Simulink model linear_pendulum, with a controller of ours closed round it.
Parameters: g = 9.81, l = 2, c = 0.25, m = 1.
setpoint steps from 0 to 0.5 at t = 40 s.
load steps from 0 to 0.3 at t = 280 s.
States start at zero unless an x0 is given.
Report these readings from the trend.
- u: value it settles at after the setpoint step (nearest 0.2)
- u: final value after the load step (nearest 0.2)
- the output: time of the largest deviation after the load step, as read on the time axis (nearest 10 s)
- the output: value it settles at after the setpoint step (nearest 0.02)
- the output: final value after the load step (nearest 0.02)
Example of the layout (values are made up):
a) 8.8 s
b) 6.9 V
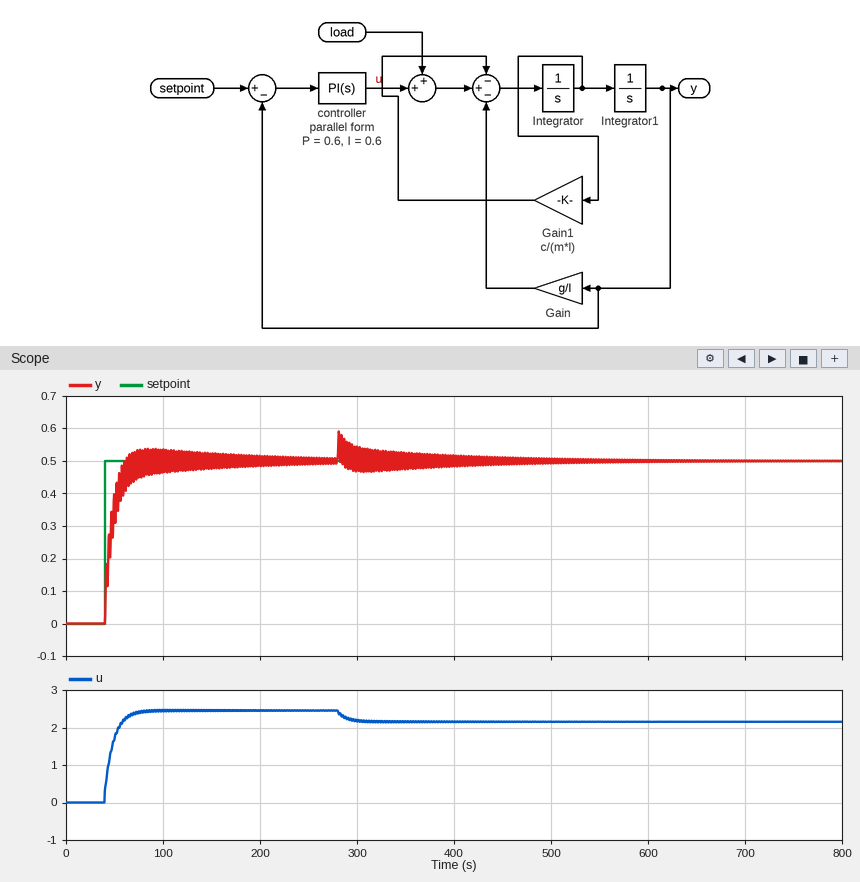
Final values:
a) 2.4
b) 2.2
c) 280 s
d) 0.50
e) 0.50
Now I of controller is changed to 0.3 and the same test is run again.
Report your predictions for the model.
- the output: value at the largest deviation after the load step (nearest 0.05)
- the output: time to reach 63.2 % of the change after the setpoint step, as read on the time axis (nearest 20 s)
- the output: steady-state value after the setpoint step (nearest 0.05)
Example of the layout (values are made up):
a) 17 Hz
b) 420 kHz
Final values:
a) 0.60
b) 60 s
c) 0.50
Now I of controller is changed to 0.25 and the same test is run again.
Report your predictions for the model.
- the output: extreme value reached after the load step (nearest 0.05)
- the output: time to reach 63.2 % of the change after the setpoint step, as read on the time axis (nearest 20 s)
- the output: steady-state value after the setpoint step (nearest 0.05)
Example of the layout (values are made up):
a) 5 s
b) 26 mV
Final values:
a) 0.60
b) 60 s
c) 0.50
